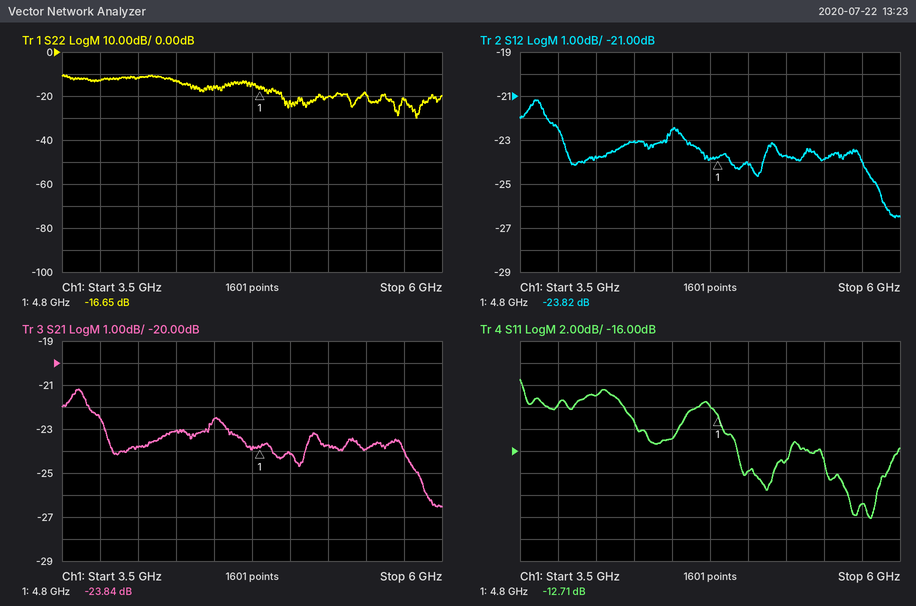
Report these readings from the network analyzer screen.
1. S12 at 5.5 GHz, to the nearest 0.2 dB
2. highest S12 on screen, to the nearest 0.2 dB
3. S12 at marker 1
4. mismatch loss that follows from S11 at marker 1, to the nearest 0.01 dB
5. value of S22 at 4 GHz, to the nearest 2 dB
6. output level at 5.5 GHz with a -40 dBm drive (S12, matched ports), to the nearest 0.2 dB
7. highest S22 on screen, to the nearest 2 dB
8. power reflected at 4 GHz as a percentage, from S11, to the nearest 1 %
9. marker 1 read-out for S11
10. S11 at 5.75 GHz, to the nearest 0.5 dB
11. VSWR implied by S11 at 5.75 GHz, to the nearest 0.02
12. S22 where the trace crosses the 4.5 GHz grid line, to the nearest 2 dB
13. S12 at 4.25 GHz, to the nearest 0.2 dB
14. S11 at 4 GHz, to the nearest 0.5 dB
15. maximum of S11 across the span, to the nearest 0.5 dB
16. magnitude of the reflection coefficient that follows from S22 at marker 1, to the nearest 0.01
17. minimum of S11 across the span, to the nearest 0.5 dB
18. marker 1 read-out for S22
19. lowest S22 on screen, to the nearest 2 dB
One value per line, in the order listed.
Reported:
-23.8 dB
-21.2 dB
-23.82 dB
0.24 dB
-12 dB
-63.8 dBm
-10 dB
8 %
-12.71 dB
-21.0 dB
1.20
-16 dB
-23.0 dB
-11.0 dB
-9.5 dB
0.15
-22.0 dB
-16.65 dB
-30 dB
